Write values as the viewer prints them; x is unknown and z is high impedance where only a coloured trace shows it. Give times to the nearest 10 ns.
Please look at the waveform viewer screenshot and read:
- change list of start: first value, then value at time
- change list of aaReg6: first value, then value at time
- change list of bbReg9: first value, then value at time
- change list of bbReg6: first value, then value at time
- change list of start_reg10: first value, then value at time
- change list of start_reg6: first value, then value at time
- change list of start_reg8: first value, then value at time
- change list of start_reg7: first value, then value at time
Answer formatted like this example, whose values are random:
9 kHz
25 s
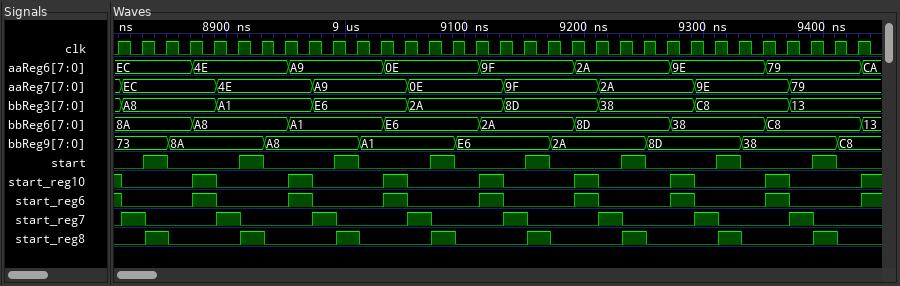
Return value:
0, 1 at 8830 ns, 0 at 8850 ns, 1 at 8910 ns, 0 at 8930 ns, 1 at 8990 ns, 0 at 9010 ns, 1 at 9070 ns, 0 at 9090 ns, 1 at 9150 ns, 0 at 9170 ns, 1 at 9230 ns, 0 at 9250 ns, 1 at 9310 ns, 0 at 9330 ns, 1 at 9390 ns, 0 at 9410 ns
EC, 4E at 8870 ns, A9 at 8950 ns, 0E at 9030 ns, 9F at 9110 ns, 2A at 9190 ns, 9E at 9270 ns, 79 at 9350 ns, CA at 9430 ns
73, 8A at 8850 ns, A8 at 8930 ns, A1 at 9010 ns, E6 at 9090 ns, 2A at 9170 ns, 8D at 9250 ns, 38 at 9330 ns, C8 at 9410 ns
8A, A8 at 8870 ns, A1 at 8950 ns, E6 at 9030 ns, 2A at 9110 ns, 8D at 9190 ns, 38 at 9270 ns, C8 at 9350 ns, 13 at 9430 ns
1, 0 at 8810 ns, 1 at 8870 ns, 0 at 8890 ns, 1 at 8950 ns, 0 at 8970 ns, 1 at 9030 ns, 0 at 9050 ns, 1 at 9110 ns, 0 at 9130 ns, 1 at 9190 ns, 0 at 9210 ns, 1 at 9270 ns, 0 at 9290 ns, 1 at 9350 ns, 0 at 9370 ns, 1 at 9430 ns
1, 0 at 8810 ns, 1 at 8870 ns, 0 at 8890 ns, 1 at 8950 ns, 0 at 8970 ns, 1 at 9030 ns, 0 at 9050 ns, 1 at 9110 ns, 0 at 9130 ns, 1 at 9190 ns, 0 at 9210 ns, 1 at 9270 ns, 0 at 9290 ns, 1 at 9350 ns, 0 at 9370 ns, 1 at 9430 ns
0, 1 at 8830 ns, 0 at 8850 ns, 1 at 8910 ns, 0 at 8930 ns, 1 at 8990 ns, 0 at 9010 ns, 1 at 9070 ns, 0 at 9090 ns, 1 at 9150 ns, 0 at 9170 ns, 1 at 9230 ns, 0 at 9250 ns, 1 at 9310 ns, 0 at 9330 ns, 1 at 9390 ns, 0 at 9410 ns
0, 1 at 8810 ns, 0 at 8830 ns, 1 at 8890 ns, 0 at 8910 ns, 1 at 8970 ns, 0 at 8990 ns, 1 at 9050 ns, 0 at 9070 ns, 1 at 9130 ns, 0 at 9150 ns, 1 at 9210 ns, 0 at 9230 ns, 1 at 9290 ns, 0 at 9310 ns, 1 at 9370 ns, 0 at 9390 ns
